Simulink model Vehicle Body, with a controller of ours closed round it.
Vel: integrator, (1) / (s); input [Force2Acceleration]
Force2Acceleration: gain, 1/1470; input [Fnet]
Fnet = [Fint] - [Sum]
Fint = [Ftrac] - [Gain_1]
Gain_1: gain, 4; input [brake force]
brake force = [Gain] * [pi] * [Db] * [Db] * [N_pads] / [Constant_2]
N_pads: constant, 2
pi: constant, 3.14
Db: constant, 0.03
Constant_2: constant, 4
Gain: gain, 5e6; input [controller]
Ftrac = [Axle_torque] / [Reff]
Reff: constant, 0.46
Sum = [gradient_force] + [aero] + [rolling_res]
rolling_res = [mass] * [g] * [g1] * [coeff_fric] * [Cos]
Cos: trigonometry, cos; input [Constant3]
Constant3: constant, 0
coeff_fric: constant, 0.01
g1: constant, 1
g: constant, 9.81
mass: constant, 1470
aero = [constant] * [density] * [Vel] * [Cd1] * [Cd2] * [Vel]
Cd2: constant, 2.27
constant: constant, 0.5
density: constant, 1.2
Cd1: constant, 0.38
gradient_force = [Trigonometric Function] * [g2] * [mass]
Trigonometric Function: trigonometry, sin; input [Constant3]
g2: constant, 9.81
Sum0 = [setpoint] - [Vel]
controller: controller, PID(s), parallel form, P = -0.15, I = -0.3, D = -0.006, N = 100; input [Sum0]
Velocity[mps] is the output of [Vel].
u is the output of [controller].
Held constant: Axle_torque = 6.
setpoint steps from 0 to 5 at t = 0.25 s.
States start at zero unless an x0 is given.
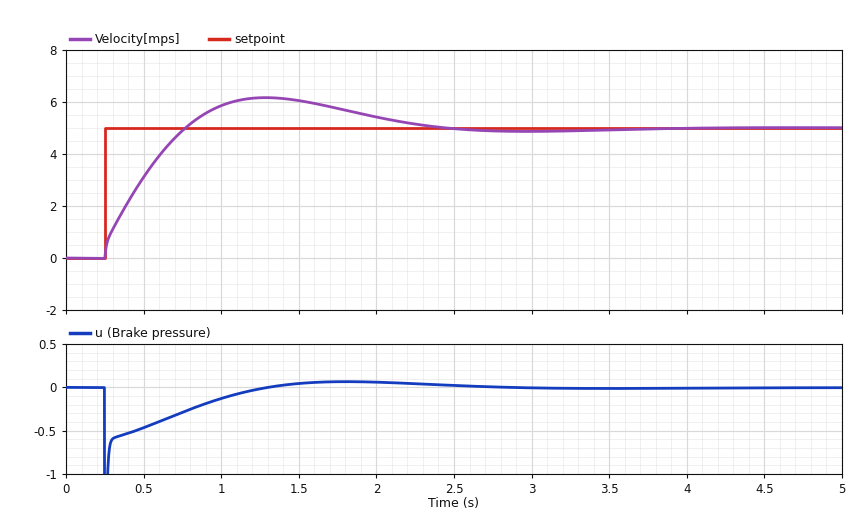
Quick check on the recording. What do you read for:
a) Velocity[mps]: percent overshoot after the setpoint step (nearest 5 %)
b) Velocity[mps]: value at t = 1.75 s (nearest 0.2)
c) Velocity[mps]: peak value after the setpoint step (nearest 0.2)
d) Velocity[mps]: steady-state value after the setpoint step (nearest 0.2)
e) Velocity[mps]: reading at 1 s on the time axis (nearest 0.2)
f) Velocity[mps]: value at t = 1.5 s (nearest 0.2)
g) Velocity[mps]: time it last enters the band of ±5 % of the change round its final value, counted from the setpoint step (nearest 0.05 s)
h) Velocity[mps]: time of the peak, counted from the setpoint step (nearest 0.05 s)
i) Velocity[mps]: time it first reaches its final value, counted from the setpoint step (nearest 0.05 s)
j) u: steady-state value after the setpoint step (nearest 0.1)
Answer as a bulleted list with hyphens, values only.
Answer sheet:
- 25 %
- 5.8
- 6.2
- 5.0
- 5.8
- 6.0
- 1.90 s
- 1.05 s
- 0.50 s
- 0.0
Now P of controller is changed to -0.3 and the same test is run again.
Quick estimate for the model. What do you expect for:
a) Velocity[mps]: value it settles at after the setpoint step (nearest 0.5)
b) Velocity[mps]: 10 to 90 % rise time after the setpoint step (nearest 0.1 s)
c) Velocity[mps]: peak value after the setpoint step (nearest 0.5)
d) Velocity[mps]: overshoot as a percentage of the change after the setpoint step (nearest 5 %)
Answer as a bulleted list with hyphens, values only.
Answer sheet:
- 5.0
- 0.3 s
- 5.5
- 10 %
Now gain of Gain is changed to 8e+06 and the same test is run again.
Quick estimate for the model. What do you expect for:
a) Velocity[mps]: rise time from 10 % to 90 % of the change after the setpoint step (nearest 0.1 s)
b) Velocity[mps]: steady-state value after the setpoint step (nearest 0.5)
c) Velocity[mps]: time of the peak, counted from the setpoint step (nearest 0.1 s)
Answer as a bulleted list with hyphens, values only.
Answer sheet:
- 0.3 s
- 5.0
- 0.8 s
